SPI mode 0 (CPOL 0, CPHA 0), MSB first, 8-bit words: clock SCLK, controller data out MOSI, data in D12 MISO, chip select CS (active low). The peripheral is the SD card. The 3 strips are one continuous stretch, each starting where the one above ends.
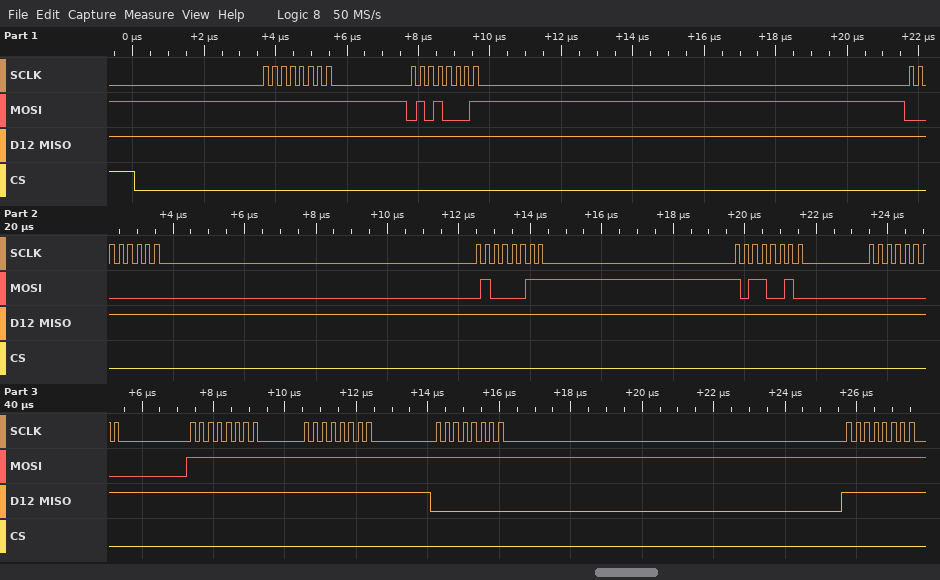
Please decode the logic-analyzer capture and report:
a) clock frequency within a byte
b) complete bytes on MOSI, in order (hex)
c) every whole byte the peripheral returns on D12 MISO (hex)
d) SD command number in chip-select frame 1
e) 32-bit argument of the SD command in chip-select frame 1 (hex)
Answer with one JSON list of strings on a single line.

["4 MHz", "0xFF 0x51 0x00 0x43 0xB2 0x00 0xFF 0xFF 0xFF 0xFF", "0xFF 0xFF 0xFF 0xFF 0xFF 0xFF 0xFF 0xFF 0x00 0xFF", "CMD17", "0x0043B200"]
